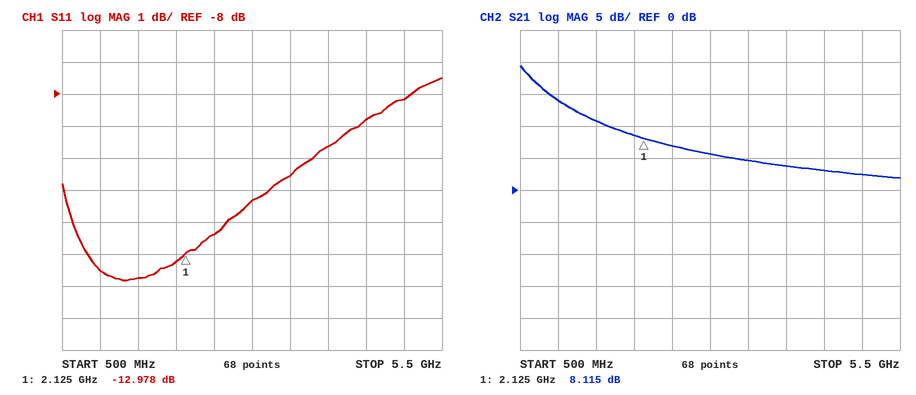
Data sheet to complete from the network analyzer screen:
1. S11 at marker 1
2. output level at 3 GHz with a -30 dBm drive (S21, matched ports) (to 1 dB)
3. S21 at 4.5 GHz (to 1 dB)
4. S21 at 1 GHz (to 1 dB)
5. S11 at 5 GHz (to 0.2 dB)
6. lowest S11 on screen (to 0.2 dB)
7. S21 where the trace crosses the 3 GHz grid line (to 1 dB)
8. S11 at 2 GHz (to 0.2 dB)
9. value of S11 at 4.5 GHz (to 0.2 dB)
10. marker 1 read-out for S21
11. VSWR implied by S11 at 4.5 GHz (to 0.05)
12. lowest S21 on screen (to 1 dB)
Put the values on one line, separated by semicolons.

-12.978 dB; -24 dBm; 3 dB; 14 dB; -8.2 dB; -13.8 dB; 6 dB; -13.2 dB; -8.8 dB; 8.115 dB; 2.15; 2 dB
